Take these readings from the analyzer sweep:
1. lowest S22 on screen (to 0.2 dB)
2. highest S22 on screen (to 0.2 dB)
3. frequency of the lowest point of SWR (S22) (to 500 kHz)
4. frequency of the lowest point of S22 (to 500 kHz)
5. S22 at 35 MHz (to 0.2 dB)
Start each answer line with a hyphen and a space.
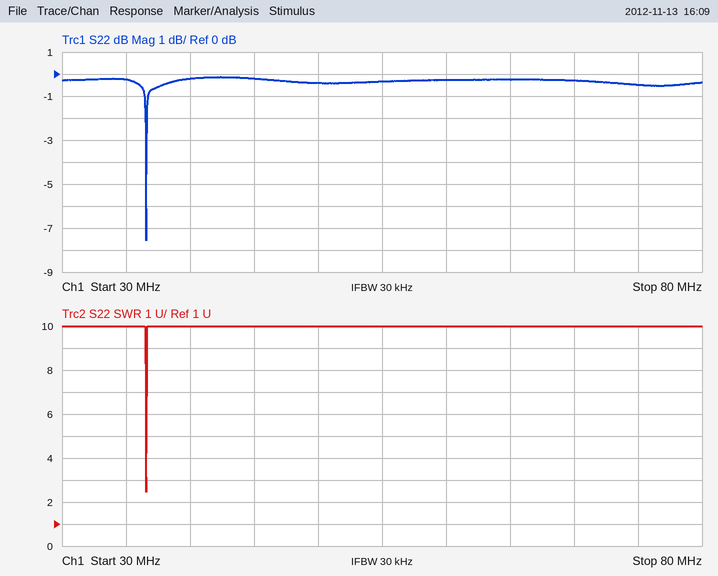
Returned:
- -7.6 dB
- -0.2 dB
- 36.5 MHz
- 36.5 MHz
- -0.2 dB
